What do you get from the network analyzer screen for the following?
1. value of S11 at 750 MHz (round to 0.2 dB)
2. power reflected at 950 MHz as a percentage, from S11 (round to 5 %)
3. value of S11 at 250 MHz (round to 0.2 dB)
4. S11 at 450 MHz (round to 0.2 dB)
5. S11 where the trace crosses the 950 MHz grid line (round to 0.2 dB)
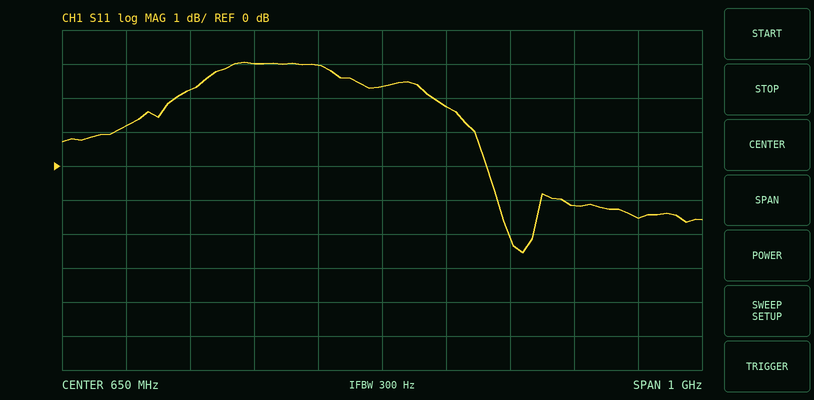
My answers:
1.8 dB
75 %
1.2 dB
3.0 dB
-1.2 dB
